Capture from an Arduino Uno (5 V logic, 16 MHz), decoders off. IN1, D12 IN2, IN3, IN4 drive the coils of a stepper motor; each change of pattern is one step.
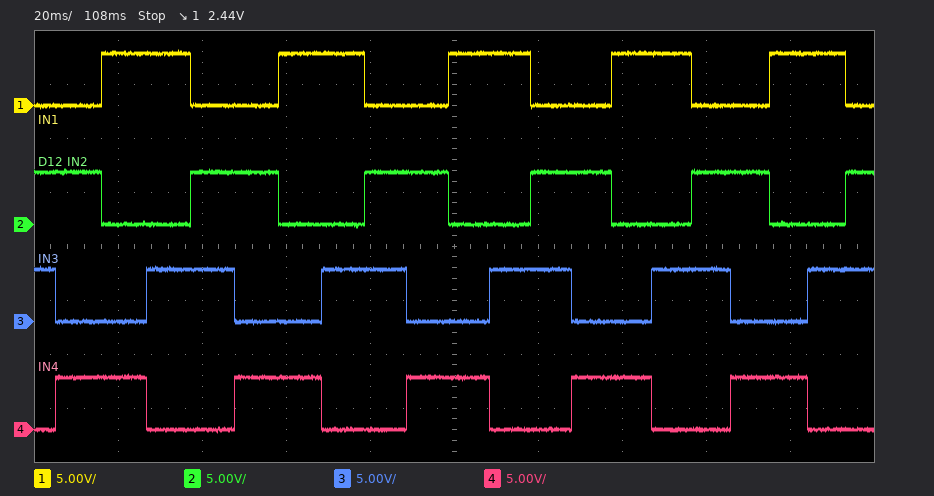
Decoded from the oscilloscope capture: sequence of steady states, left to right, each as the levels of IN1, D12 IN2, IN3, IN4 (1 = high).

0110 0101 1001 1010 0110 0101 1001 1010 0110 0101 1001 1010 0110 0101 1001 1010 0110 0101 1001 1010 0110
